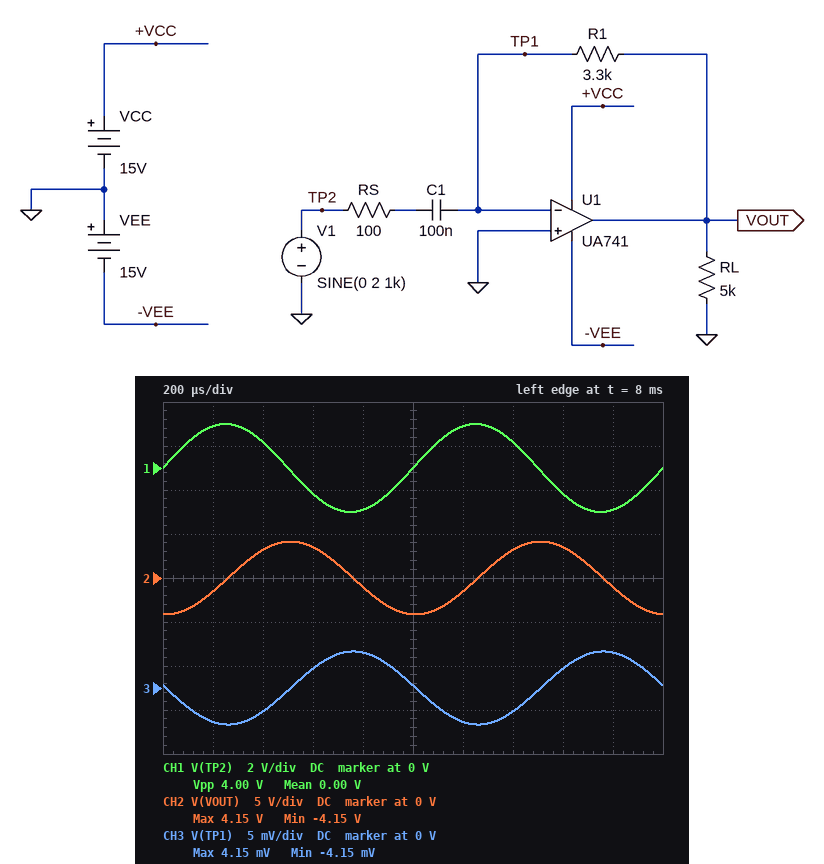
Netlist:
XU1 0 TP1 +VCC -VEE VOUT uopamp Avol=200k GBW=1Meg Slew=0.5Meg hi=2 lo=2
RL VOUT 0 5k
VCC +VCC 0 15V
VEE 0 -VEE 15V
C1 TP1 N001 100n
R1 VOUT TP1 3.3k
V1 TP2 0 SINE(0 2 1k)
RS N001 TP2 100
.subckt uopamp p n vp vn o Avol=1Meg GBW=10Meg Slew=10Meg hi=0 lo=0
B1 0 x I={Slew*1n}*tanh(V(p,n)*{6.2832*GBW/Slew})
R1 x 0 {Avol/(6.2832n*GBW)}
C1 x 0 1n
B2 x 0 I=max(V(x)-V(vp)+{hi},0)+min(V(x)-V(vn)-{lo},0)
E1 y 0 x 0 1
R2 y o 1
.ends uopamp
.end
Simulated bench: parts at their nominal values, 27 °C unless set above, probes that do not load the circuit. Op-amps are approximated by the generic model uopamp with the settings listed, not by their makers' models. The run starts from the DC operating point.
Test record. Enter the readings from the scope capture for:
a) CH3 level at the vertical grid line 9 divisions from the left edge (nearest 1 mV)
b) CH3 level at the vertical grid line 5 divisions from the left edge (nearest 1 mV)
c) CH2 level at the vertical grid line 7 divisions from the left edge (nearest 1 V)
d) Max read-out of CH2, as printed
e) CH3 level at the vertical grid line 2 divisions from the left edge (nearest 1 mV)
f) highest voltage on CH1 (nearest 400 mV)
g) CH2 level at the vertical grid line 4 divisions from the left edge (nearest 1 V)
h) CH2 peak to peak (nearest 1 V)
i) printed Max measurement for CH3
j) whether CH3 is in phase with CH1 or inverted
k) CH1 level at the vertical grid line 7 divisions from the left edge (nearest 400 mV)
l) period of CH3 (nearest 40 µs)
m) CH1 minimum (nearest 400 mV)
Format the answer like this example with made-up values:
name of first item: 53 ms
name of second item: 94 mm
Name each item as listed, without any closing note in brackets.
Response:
CH3 level at the vertical grid line 9 divisions from the left edge: 4 mV
CH3 level at the vertical grid line 5 divisions from the left edge: 0 V
CH2 level at the vertical grid line 7 divisions from the left edge: 3 V
Max read-out of CH2, as printed: 4.15 V
CH3 level at the vertical grid line 2 divisions from the left edge: -3 mV
highest voltage on CH1: 2.0 V
CH2 level at the vertical grid line 4 divisions from the left edge: -1 V
CH2 peak to peak: 8 V
printed Max measurement for CH3: 4.15 mV
whether CH3 is in phase with CH1 or inverted: inverted
CH1 level at the vertical grid line 7 divisions from the left edge: 1.2 V
period of CH3: 1.00 ms
CH1 minimum: -2.0 V
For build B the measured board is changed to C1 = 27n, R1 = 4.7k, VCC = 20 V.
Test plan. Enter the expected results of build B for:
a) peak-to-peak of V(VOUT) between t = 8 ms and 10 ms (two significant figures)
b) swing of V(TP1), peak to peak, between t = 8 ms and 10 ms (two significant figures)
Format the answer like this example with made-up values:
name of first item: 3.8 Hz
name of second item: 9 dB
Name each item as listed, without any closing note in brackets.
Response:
peak-to-peak of V(VOUT) between t = 8 ms and 10 ms: 3.2 V
swing of V(TP1), peak to peak, between t = 8 ms and 10 ms: 3.2 mV
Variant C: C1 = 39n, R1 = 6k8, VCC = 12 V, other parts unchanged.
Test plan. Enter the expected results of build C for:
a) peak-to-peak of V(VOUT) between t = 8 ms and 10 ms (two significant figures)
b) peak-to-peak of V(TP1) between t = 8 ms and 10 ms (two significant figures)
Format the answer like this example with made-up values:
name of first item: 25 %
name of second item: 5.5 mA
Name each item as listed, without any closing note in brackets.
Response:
peak-to-peak of V(VOUT) between t = 8 ms and 10 ms: 6.7 V
peak-to-peak of V(TP1) between t = 8 ms and 10 ms: 6.7 mV
